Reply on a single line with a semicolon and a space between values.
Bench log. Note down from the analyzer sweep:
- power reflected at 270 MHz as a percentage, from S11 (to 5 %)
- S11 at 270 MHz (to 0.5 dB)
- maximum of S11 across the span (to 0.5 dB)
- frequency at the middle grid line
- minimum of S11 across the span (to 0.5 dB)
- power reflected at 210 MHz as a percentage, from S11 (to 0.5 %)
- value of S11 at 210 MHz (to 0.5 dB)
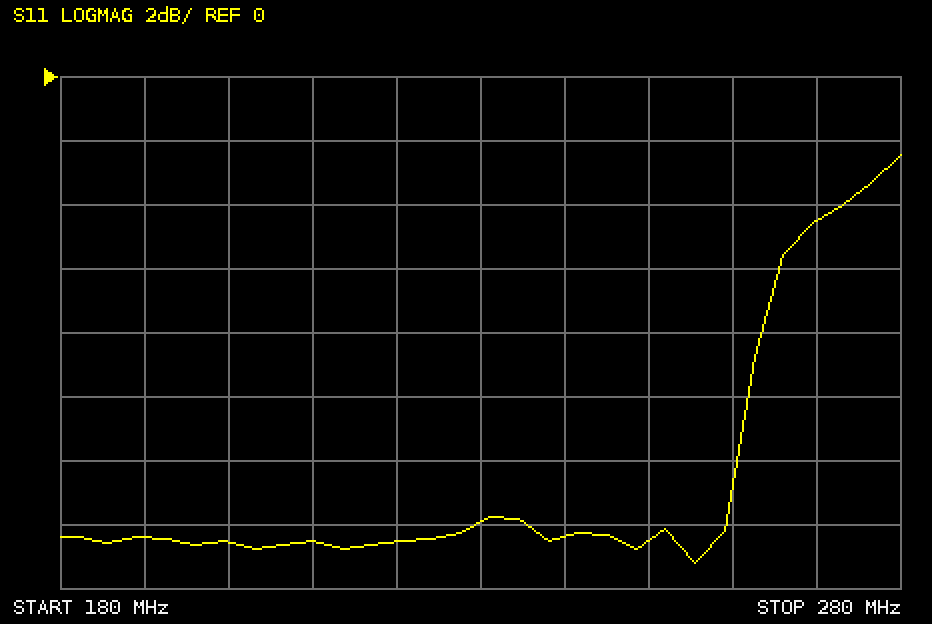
35 %; -4.5 dB; -2.5 dB; 230 MHz; -15.0 dB; 3.5 %; -14.5 dB
